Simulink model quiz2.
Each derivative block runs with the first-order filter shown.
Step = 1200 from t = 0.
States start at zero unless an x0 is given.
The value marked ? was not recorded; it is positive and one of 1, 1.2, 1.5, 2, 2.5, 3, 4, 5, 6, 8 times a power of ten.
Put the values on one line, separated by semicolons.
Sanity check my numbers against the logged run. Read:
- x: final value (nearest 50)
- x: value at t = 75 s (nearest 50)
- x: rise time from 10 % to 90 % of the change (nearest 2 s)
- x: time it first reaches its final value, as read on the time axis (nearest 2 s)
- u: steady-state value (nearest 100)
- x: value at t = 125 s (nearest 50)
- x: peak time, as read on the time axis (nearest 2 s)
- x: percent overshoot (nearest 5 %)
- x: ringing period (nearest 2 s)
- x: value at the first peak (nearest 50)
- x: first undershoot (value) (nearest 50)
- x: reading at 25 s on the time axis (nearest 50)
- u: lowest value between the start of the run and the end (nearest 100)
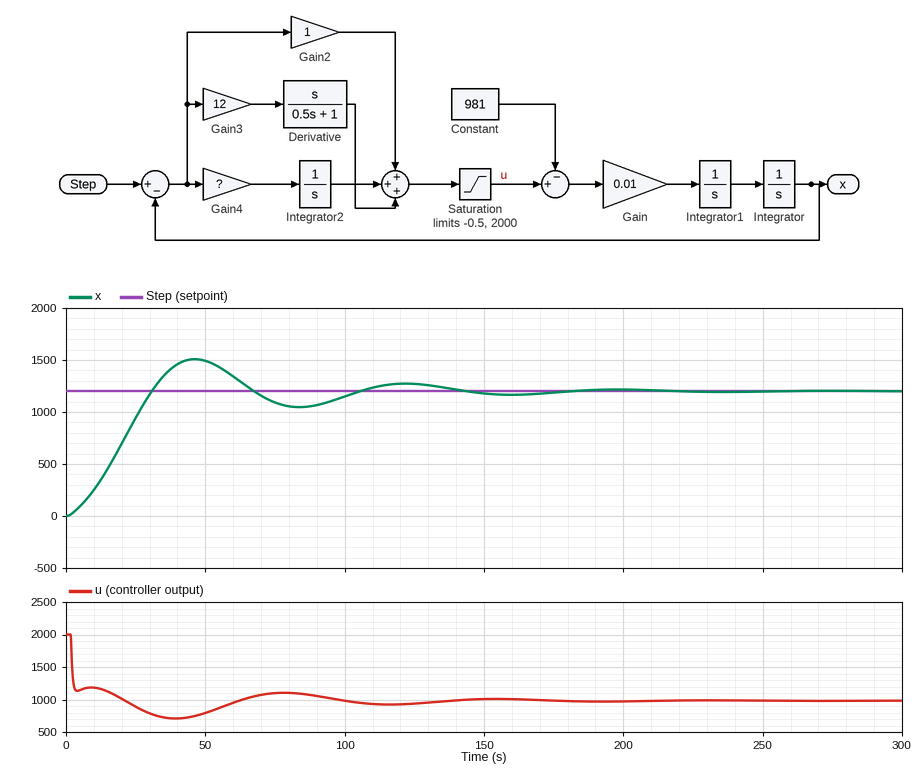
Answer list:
1200; 1100; 22 s; 30 s; 1000; 1250; 46 s; 25 %; 76 s; 1500; 1050; 950; 700
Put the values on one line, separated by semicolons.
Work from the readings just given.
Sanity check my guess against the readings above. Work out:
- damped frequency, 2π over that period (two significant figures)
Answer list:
0.083 rad/s
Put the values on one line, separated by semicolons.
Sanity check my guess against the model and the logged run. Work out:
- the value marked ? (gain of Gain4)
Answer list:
0.06
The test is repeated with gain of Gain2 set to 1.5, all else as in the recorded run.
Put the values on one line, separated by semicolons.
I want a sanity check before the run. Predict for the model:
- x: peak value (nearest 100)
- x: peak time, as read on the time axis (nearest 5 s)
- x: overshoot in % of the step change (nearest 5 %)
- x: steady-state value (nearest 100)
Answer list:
1300; 35 s; 10 %; 1200
